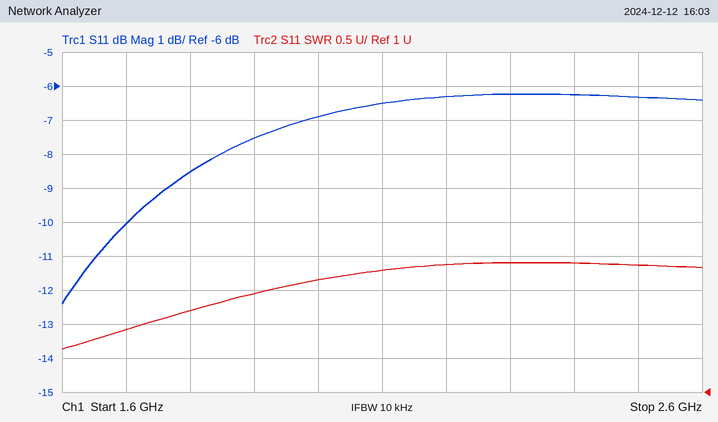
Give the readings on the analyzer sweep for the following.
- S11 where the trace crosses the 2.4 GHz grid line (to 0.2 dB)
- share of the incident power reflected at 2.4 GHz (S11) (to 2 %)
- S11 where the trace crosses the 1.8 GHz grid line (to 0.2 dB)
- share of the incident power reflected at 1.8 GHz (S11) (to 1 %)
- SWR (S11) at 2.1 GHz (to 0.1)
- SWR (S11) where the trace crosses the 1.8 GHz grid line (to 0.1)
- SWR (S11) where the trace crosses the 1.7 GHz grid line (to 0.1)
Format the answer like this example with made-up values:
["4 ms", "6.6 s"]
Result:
["-6.2 dB", "24 %", "-8.6 dB", "14 %", "2.8", "2.2", "1.9"]
